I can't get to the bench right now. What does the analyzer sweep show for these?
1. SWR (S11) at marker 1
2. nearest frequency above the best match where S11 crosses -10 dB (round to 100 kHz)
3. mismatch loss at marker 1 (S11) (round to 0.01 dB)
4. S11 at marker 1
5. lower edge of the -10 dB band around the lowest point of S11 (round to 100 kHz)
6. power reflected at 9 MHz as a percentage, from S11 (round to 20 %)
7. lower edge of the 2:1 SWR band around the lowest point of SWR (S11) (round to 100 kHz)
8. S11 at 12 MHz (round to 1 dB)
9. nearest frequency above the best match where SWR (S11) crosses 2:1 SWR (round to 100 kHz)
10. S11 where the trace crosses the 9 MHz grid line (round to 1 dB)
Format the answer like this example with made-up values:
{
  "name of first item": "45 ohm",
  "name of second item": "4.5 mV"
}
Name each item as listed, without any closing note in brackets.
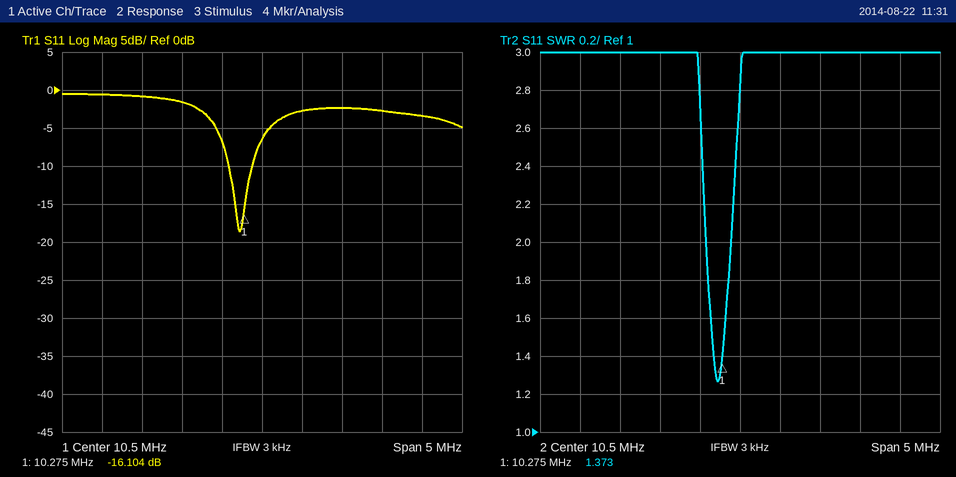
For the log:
{
  "SWR (S11) at marker 1": "1.373",
  "nearest frequency above the best match where S11 crosses -10 dB": "10.4 MHz",
  "mismatch loss at marker 1 (S11)": "0.11 dB",
  "S11 at marker 1": "-16.104 dB",
  "lower edge of the -10 dB band around the lowest point of S11": "10.1 MHz",
  "power reflected at 9 MHz as a percentage, from S11": "80 %",
  "lower edge of the 2:1 SWR band around the lowest point of SWR (S11)": "10.1 MHz",
  "S11 at 12 MHz": "-3 dB",
  "nearest frequency above the best match where SWR (S11) crosses 2:1 SWR": "10.4 MHz",
  "S11 where the trace crosses the 9 MHz grid line": "-1 dB"
}
